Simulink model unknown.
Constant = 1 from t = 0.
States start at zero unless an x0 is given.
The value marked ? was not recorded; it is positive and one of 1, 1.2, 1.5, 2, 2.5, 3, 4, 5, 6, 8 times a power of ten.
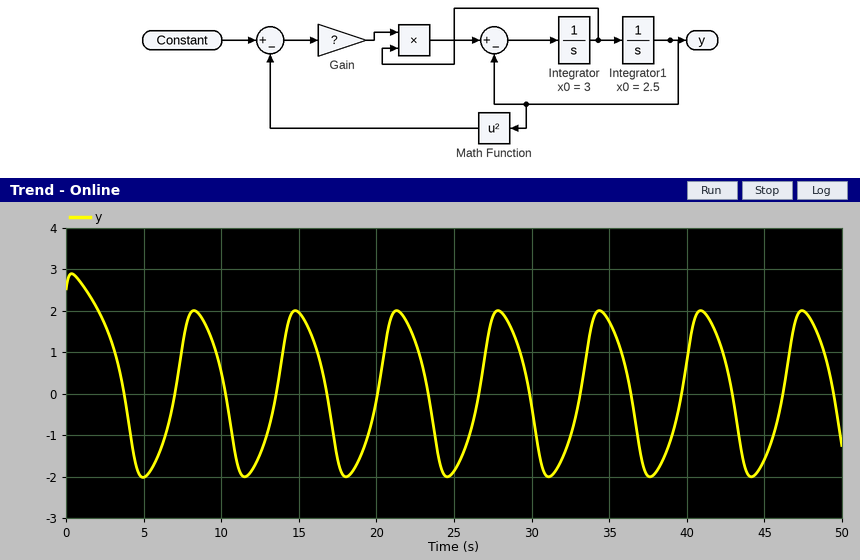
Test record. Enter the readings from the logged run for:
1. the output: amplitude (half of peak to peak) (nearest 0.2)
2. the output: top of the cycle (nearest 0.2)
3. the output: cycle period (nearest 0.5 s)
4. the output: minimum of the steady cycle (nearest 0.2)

2.0
2.0
6.5 s
-2.0
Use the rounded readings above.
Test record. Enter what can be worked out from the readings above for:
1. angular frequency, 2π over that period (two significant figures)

0.97 rad/s
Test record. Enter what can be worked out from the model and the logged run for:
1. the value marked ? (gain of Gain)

0.8
